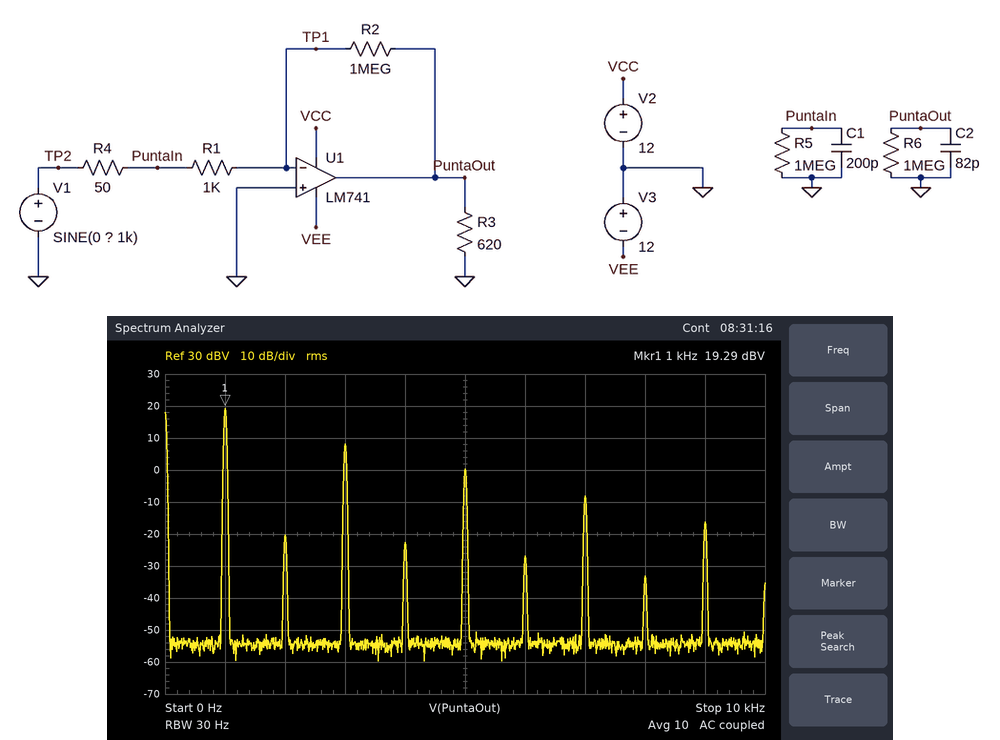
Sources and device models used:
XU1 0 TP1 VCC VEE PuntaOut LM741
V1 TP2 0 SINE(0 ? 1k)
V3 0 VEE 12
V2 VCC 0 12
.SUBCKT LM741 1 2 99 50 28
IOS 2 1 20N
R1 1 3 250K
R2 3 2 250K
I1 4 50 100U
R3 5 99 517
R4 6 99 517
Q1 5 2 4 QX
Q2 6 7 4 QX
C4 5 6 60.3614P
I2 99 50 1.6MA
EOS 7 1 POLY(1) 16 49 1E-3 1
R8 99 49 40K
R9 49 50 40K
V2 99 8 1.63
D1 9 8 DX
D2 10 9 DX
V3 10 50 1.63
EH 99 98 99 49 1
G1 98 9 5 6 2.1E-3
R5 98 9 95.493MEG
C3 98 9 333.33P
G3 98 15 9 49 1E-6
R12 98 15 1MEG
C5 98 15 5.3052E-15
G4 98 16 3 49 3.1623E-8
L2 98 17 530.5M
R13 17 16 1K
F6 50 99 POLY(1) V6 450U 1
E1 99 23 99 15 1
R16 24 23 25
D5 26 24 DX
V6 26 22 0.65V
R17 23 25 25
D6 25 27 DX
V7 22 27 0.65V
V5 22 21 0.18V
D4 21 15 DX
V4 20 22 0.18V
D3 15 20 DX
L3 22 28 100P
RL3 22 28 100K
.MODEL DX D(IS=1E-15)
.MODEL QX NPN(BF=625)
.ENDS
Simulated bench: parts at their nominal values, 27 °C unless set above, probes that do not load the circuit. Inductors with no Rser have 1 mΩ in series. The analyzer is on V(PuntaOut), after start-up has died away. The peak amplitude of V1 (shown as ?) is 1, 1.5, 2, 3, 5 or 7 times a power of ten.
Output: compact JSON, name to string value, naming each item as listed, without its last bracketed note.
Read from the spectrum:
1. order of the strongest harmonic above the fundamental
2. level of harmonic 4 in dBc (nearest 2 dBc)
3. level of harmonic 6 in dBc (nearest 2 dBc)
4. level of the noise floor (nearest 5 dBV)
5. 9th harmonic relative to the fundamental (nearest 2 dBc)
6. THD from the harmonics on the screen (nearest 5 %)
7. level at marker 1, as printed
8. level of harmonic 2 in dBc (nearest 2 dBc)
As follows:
{"order of the strongest harmonic above the fundamental": "3", "level of harmonic 4 in dBc": "-42 dBc", "level of harmonic 6 in dBc": "-46 dBc", "level of the noise floor": "-55 dBV", "9th harmonic relative to the fundamental": "-36 dBc", "THD from the harmonics on the screen": "30 %", "level at marker 1, as printed": "19.29 dBV", "level of harmonic 2 in dBc": "-40 dBc"}
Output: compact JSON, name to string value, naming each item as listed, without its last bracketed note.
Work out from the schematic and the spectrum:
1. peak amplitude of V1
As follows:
{"peak amplitude of V1": "100 mV"}
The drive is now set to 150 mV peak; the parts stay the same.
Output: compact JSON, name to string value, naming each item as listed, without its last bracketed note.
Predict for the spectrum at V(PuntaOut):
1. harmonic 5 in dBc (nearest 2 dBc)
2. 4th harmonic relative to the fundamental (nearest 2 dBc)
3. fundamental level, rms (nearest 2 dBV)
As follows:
{"harmonic 5 in dBc": "-18 dBc", "4th harmonic relative to the fundamental": "-44 dBc", "fundamental level, rms": "20 dBV"}
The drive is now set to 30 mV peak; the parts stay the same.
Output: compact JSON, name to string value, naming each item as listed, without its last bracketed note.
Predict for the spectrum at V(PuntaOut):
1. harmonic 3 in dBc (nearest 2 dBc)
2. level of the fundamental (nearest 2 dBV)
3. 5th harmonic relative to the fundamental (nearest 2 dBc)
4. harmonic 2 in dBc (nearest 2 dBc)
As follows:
{"harmonic 3 in dBc": "-16 dBc", "level of the fundamental": "18 dBV", "5th harmonic relative to the fundamental": "-32 dBc", "harmonic 2 in dBc": "-30 dBc"}
